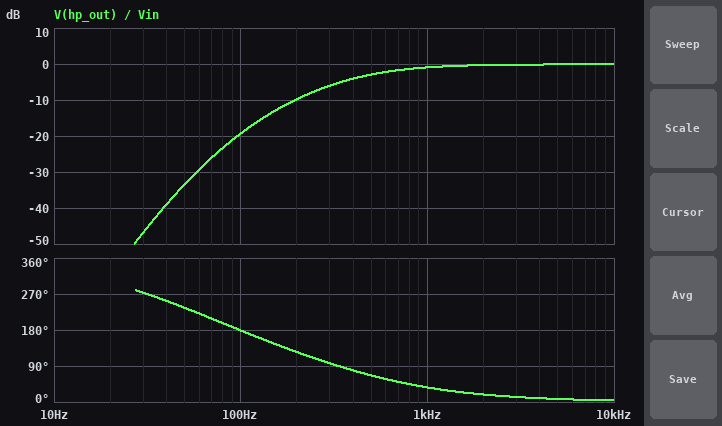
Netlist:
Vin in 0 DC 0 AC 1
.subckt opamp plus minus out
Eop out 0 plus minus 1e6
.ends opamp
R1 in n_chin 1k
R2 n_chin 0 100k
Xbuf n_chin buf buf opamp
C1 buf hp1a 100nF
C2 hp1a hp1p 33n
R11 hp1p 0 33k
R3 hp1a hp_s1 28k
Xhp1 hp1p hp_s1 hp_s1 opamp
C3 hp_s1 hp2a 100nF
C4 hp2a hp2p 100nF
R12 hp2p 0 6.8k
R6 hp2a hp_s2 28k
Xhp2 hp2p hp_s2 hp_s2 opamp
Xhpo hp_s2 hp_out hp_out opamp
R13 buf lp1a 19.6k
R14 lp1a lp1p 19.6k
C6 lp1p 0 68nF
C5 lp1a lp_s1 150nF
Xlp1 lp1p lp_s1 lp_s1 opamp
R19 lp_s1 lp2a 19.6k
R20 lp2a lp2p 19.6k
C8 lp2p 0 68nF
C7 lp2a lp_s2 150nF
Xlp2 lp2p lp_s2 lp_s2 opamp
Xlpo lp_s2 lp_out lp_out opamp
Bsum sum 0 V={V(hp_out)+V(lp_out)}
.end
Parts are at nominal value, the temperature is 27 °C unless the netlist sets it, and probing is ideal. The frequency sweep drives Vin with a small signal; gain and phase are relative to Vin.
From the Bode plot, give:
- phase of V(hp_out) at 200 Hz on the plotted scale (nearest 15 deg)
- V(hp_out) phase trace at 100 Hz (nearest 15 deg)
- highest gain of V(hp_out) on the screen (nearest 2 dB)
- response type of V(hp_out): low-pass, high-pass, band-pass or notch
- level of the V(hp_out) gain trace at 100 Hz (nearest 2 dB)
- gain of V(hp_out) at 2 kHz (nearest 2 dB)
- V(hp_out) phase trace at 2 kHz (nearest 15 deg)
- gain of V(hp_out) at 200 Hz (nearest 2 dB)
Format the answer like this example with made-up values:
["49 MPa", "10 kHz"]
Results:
["120 deg", "180 deg", "0 dB", "high-pass", "-20 dB", "0 dB", "15 deg", "-10 dB"]
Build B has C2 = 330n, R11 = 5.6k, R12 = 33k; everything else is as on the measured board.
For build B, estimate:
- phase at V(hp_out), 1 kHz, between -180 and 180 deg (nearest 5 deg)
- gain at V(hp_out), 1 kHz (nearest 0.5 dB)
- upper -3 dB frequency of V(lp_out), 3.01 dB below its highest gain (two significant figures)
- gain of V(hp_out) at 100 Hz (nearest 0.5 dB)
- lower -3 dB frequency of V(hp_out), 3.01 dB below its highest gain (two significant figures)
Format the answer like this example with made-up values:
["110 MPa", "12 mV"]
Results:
["25 deg", "-0.5 dB", "69 Hz", "-13.0 dB", "370 Hz"]
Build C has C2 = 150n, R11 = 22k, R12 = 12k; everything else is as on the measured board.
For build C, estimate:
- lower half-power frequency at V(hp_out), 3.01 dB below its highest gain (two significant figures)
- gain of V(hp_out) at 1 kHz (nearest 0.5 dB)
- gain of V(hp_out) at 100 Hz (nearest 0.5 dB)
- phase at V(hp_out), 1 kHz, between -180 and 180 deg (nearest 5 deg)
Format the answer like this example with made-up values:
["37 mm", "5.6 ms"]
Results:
["270 Hz", "-0.5 dB", "-11.5 dB", "20 deg"]
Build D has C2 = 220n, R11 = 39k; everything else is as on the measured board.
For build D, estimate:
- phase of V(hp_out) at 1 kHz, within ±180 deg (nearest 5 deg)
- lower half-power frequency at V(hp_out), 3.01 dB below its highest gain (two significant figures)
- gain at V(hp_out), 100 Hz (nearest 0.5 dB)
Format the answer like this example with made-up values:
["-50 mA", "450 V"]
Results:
["30 deg", "440 Hz", "-14.0 dB"]
